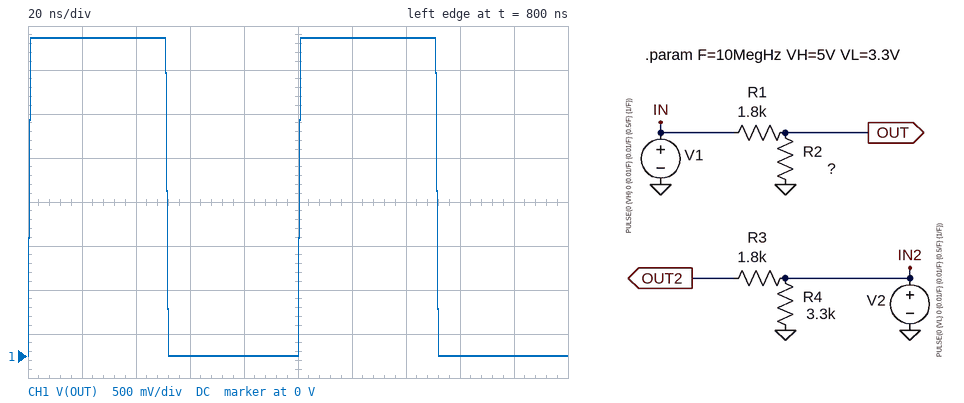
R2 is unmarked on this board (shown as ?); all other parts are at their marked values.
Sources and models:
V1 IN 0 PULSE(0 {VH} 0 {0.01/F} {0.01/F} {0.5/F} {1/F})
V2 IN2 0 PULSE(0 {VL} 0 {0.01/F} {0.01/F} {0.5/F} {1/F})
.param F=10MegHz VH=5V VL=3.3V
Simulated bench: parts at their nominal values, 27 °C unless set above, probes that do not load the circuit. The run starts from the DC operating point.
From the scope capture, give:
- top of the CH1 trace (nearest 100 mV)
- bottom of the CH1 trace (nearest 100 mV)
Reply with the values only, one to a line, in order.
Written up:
3.6 V
0 V
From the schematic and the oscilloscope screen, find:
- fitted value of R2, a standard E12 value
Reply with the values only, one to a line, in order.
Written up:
4.7 kΩ
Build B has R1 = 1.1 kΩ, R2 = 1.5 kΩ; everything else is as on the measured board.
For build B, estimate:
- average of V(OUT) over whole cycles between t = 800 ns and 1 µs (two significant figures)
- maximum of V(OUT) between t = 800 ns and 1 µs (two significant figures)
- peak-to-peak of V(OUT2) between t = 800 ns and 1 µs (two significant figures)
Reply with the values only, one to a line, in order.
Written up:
1.5 V
2.9 V
3.3 V
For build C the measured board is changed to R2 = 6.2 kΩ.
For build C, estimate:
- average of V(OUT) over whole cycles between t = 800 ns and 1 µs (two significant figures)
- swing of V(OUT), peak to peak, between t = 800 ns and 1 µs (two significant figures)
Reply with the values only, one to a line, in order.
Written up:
2.0 V
3.9 V
